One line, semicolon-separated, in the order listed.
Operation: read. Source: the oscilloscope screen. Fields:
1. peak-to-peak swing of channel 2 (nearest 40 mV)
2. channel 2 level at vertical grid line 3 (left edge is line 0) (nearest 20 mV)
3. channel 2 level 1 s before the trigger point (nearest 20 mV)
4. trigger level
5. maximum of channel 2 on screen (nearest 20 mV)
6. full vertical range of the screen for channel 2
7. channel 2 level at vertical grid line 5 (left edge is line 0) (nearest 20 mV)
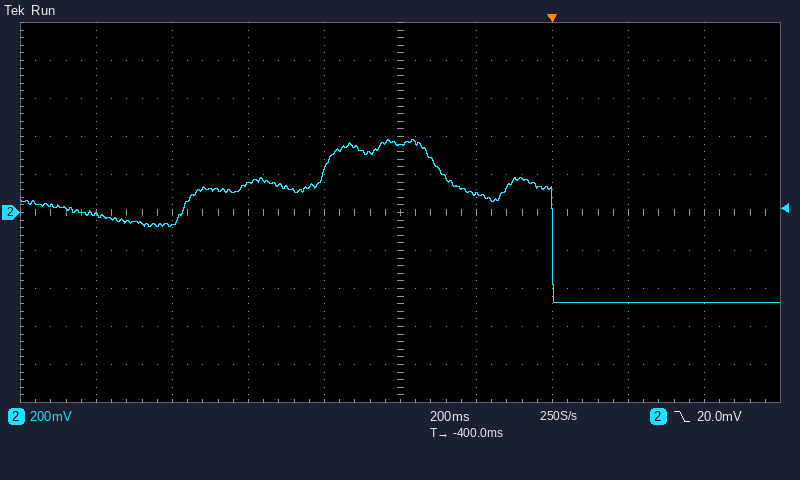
840 mV; 140 mV; -60 mV; 20.0 mV; 380 mV; 2 V; 360 mV
